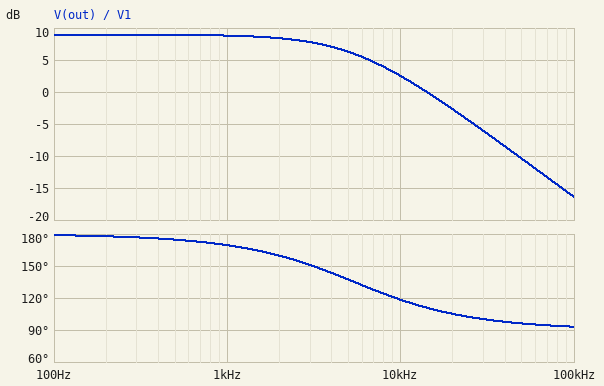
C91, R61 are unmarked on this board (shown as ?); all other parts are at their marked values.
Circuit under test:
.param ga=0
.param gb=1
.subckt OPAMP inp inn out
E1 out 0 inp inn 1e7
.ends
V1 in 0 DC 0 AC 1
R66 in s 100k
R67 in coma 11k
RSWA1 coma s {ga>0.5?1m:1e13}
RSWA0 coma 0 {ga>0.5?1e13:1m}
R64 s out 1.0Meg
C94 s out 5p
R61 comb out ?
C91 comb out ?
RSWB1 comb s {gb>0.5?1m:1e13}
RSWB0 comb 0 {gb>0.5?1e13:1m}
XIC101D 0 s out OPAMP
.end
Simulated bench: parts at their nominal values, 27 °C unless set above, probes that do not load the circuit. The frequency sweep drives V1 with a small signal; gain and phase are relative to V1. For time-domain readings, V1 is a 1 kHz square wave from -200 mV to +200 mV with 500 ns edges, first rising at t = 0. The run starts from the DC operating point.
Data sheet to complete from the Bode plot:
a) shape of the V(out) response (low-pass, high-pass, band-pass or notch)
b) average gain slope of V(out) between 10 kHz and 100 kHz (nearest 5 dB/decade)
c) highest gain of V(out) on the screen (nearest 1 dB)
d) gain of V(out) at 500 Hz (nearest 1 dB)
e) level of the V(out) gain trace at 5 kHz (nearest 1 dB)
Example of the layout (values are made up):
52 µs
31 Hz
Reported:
low-pass
-20 dB/decade
9 dB
9 dB
6 dB
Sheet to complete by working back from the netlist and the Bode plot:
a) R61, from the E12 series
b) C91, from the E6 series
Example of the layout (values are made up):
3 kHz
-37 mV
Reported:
390 kΩ
100 pF
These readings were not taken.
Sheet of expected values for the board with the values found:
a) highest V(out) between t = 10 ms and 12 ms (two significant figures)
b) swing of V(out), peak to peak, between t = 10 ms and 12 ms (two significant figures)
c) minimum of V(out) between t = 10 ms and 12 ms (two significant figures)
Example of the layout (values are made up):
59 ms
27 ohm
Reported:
560 mV
1.1 V
-560 mV
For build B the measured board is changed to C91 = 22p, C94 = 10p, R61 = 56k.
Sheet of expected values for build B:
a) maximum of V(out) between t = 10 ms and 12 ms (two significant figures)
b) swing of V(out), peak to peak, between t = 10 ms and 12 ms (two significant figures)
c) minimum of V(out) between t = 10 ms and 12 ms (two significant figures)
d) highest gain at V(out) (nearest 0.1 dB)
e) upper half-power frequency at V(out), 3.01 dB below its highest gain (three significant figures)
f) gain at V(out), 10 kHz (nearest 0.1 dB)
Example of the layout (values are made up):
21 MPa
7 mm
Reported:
110 mV
210 mV
-110 mV
-5.5 dB
93.8 kHz
-5.6 dB
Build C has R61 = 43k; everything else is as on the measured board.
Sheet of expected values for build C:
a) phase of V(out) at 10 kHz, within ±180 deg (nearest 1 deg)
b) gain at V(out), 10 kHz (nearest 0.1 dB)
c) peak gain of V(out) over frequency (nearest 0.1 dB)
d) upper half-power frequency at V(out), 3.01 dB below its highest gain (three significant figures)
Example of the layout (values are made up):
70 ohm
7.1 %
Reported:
165 deg
-8.0 dB
-7.7 dB
36.8 kHz
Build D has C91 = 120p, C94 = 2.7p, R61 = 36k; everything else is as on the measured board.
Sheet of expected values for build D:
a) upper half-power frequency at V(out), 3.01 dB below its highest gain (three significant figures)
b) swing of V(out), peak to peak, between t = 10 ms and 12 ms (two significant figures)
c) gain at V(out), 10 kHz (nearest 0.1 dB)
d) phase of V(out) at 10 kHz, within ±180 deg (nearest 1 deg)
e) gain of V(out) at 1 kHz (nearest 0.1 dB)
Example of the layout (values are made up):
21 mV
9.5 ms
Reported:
37.3 kHz
140 mV
-9.5 dB
165 deg
-9.2 dB
